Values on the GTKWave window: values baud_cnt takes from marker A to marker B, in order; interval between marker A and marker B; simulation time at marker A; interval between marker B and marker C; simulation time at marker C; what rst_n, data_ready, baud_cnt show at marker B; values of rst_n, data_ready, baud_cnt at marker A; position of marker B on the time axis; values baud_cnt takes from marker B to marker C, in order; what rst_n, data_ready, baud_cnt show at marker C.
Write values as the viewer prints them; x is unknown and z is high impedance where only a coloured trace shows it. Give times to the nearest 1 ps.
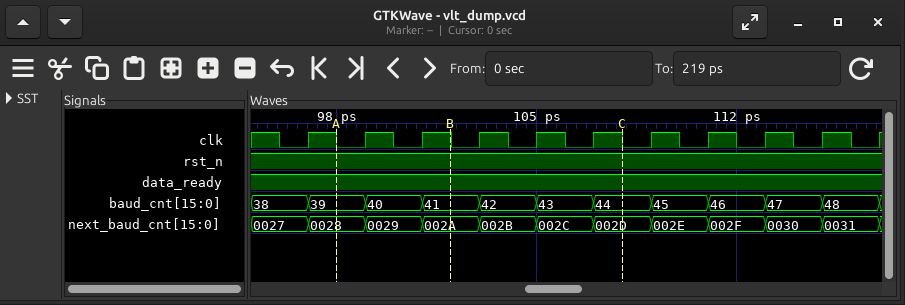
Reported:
39, 40, 41
4 ps
98 ps
6 ps
108 ps
rst_n=1, data_ready=1, baud_cnt=41
rst_n=1, data_ready=1, baud_cnt=39
102 ps
41, 42, 43, 44
rst_n=1, data_ready=1, baud_cnt=44
